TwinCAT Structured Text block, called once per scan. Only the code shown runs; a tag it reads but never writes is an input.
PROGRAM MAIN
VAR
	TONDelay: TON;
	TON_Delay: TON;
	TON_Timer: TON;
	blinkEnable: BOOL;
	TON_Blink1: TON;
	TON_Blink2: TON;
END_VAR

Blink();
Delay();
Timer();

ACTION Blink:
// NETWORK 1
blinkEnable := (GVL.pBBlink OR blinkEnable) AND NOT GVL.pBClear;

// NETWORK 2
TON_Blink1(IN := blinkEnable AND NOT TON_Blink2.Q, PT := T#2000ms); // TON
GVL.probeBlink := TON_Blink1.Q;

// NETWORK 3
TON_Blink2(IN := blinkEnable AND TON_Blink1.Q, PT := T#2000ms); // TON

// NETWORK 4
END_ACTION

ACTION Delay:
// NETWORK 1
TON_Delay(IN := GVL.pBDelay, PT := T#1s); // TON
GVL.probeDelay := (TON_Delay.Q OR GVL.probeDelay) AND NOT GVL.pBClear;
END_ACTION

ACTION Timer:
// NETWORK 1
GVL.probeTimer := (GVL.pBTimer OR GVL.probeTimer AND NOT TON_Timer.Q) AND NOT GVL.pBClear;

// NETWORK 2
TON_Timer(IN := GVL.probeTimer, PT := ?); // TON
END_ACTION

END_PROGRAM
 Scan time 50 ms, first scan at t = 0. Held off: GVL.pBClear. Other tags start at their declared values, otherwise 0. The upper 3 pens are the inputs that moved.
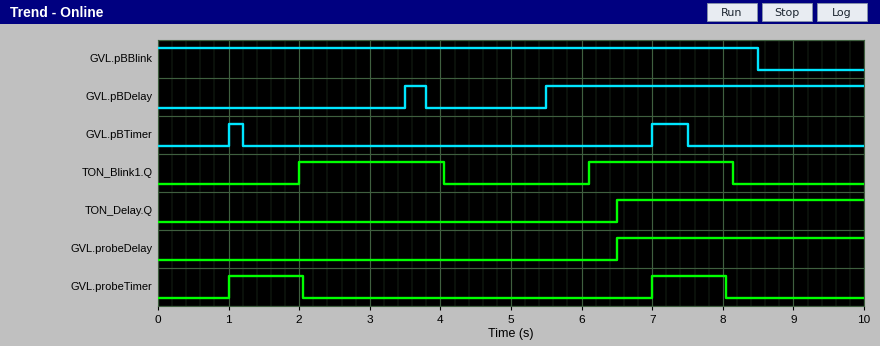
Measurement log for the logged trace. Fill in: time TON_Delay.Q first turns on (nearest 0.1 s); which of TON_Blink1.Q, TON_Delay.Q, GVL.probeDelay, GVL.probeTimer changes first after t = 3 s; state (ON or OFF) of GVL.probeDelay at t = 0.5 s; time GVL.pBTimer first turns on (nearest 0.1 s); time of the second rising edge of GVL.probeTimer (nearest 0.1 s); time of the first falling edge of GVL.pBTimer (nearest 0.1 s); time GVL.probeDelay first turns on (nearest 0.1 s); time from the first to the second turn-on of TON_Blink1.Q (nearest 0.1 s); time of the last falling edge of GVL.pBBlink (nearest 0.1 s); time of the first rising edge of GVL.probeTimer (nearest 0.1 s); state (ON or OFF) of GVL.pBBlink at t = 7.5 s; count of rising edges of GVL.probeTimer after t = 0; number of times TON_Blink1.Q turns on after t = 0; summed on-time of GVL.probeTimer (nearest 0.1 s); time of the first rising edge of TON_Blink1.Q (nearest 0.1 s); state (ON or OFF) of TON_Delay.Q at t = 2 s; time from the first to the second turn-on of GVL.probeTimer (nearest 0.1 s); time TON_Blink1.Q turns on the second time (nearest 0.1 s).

6.5 s
TON_Blink1.Q
OFF
1.0 s
7.0 s
1.2 s
6.5 s
4.1 s
8.5 s
1.0 s
ON
2
2
2.1 s
2.0 s
OFF
6.0 s
6.1 s
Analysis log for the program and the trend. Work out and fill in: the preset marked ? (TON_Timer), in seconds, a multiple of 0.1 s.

1.0 s
